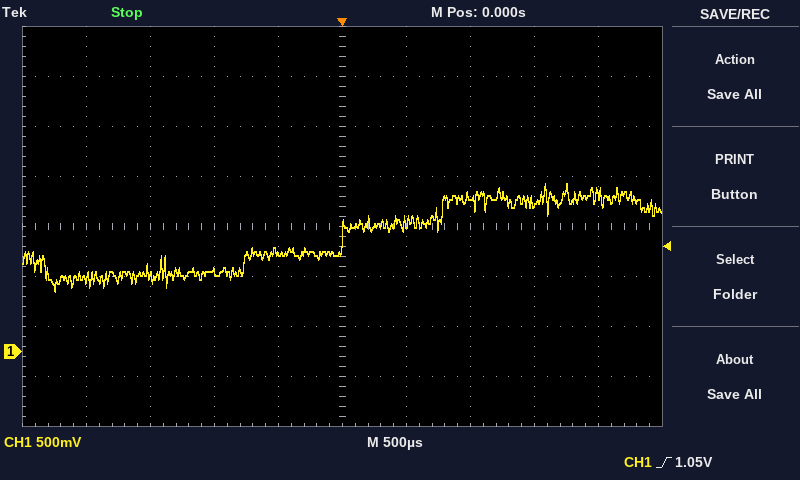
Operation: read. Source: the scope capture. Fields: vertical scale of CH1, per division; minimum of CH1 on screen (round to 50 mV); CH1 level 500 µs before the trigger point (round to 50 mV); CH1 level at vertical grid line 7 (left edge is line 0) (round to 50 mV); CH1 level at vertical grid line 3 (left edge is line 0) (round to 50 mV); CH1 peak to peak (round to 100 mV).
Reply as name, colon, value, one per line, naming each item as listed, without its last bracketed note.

vertical scale of CH1, per division: 500 mV
minimum of CH1 on screen: 600 mV
CH1 level 500 µs before the trigger point: 1.00 V
CH1 level at vertical grid line 7 (left edge is line 0): 1.55 V
CH1 level at vertical grid line 3 (left edge is line 0): 800 mV
CH1 peak to peak: 1.10 V
